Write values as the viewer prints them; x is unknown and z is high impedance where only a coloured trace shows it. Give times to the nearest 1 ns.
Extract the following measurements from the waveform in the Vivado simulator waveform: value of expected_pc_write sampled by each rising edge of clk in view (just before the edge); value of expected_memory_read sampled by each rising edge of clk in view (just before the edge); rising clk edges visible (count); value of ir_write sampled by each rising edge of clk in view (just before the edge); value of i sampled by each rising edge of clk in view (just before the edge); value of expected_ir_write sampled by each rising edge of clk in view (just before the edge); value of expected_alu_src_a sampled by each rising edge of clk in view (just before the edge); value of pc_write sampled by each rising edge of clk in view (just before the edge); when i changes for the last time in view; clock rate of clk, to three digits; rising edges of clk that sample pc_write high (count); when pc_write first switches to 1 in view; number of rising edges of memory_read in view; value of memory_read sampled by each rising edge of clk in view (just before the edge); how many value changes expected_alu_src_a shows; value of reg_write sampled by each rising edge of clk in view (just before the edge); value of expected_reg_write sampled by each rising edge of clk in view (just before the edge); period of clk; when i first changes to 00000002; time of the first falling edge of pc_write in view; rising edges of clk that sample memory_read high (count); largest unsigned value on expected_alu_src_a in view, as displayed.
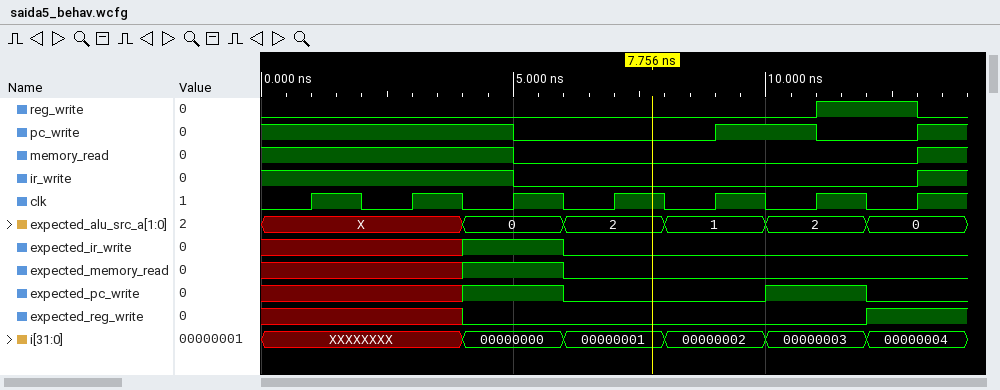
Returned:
x x 1 0 0 1 0
x x 1 0 0 0 0
7
1 1 1 0 0 0 0
XXXXXXXX, XXXXXXXX, 00000000, 00000001, 00000002, 00000003, 00000004
x x 1 0 0 0 0
X, X, 0, 2, 1, 2, 0
1 1 1 0 0 1 0
12 ns
500 MHz
4
9 ns
1
1 1 1 0 0 0 0
5
0 0 0 0 0 0 1
x x 0 0 0 0 1
2 ns
8 ns
5 ns
3
2
